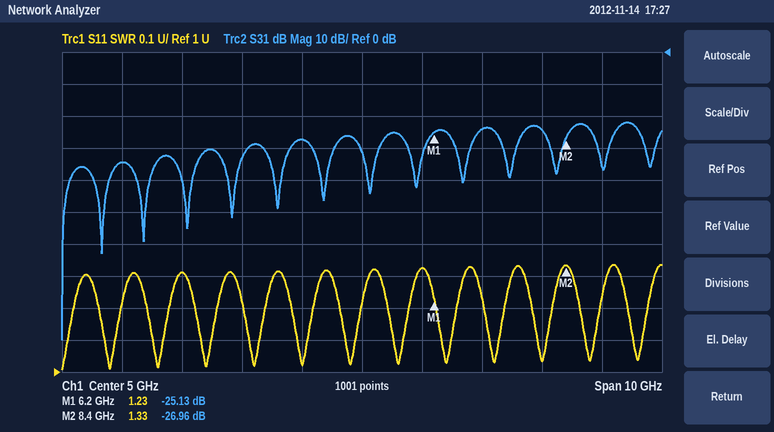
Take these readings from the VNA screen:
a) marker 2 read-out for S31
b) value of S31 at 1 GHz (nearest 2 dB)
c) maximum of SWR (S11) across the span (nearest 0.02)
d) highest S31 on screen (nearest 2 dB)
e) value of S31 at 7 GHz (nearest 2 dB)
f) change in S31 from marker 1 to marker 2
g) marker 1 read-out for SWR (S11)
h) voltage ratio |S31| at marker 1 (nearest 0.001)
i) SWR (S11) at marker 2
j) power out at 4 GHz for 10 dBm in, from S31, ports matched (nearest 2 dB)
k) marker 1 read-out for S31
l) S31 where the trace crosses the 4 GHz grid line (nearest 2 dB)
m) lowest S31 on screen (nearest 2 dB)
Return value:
-26.96 dB
-34 dB
1.34
-22 dB
-24 dB
-1.83 dB
1.23
0.055
1.33
-18 dBm
-25.13 dB
-28 dB
-90 dB
